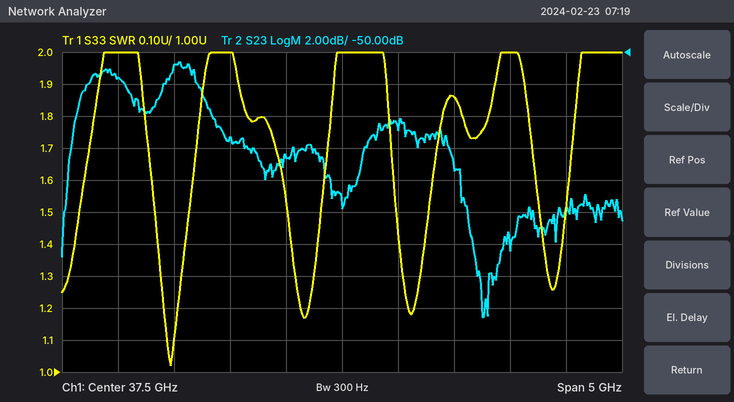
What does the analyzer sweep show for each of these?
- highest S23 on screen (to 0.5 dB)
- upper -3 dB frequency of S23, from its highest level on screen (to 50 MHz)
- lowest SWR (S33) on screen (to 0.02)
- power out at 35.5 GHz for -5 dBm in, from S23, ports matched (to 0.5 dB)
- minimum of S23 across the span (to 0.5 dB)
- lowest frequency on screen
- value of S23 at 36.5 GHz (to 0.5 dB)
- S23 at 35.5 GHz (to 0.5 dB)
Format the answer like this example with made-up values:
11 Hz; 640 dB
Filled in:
-50.5 dB; 36.30 GHz; 1.02; -56.5 dBm; -66.5 dB; 35 GHz; -55.5 dB; -51.5 dB
